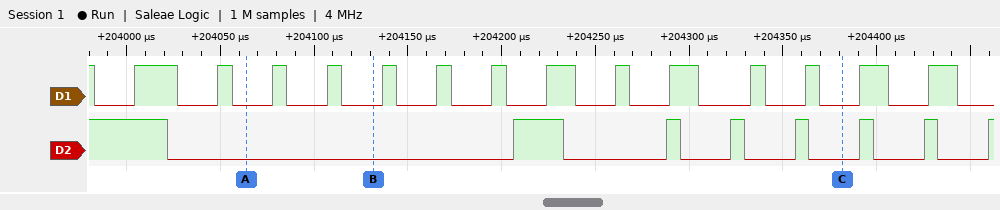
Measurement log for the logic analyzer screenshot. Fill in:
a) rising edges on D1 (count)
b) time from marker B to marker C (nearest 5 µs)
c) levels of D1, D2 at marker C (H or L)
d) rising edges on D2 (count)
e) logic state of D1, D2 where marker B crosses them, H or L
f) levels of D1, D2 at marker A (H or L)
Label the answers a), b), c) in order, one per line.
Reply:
a) 14
b) 250 µs
c) D1=L, D2=L
d) 7
e) D1=L, D2=L
f) D1=L, D2=L
